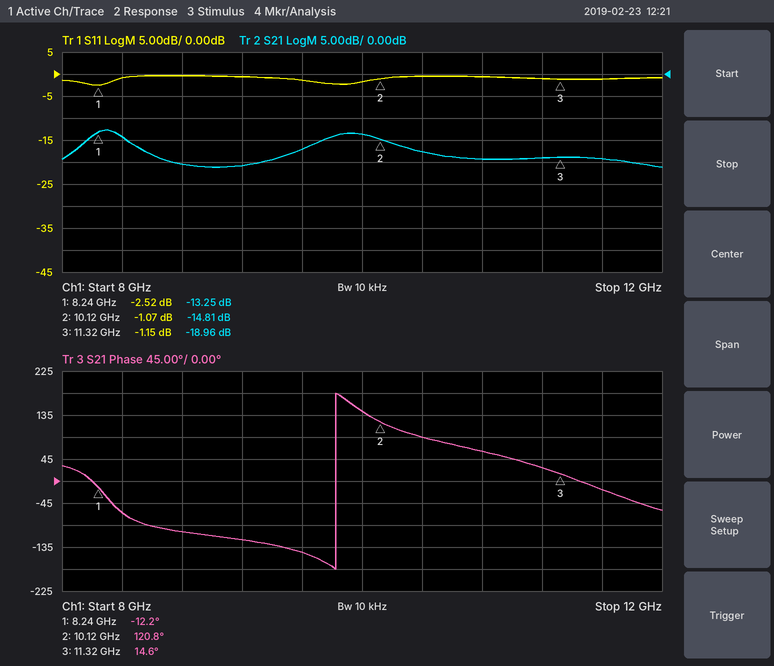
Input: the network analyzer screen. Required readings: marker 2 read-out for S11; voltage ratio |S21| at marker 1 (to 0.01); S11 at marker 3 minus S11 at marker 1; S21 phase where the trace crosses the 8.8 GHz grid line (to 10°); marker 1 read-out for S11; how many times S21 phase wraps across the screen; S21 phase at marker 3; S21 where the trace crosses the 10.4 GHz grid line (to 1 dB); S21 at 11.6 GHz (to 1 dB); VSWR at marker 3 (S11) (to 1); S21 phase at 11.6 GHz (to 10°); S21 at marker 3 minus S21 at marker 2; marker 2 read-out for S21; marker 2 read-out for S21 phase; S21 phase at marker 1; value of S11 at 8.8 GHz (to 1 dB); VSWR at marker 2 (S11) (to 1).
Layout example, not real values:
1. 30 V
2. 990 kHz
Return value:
1. -1.07 dB
2. 0.22
3. 1.37 dB
4. -100°
5. -2.52 dB
6. 1
7. 14.6°
8. -18 dB
9. -19 dB
10. 15
11. -20°
12. -4.15 dB
13. -14.81 dB
14. 120.8°
15. -12.2°
16. 0 dB
17. 16
